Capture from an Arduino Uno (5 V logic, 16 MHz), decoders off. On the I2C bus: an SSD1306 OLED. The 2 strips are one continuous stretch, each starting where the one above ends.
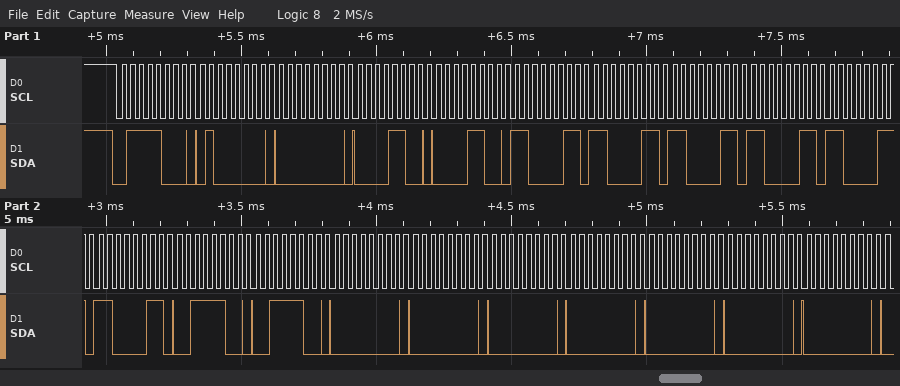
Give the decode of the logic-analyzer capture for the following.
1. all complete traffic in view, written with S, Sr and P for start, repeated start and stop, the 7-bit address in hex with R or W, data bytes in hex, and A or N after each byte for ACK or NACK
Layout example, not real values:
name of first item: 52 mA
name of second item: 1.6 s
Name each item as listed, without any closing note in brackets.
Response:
all complete traffic in view, written with S, Sr and P for start, repeated start and stop, the 7-bit address in hex with R or W, data bytes in hex, and A or N after each byte for ACK or NACK: S 3CW A 40 A 00 A 0C A 0C A C3 A C3 A C3 A C3 A C3 A C3 A 3C A 3C A 00 A 00 A 00 A 00 A 00 A 00 A 00 A
